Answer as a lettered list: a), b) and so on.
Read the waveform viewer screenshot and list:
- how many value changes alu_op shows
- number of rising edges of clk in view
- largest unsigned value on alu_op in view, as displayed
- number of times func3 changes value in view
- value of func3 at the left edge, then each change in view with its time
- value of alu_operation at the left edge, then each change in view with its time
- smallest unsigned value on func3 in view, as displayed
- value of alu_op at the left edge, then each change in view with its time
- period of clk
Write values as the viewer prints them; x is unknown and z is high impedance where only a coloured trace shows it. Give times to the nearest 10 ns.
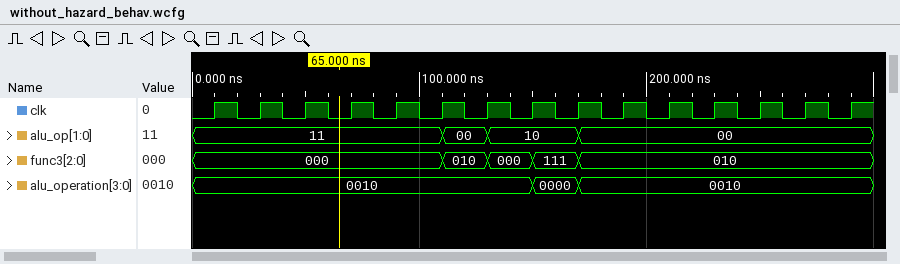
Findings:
a) 3
b) 15
c) 11
d) 4
e) 000, 010 at 110 ns, 000 at 130 ns, 111 at 150 ns, 010 at 170 ns
f) 0010, 0000 at 150 ns, 0010 at 170 ns
g) 000
h) 11, 00 at 110 ns, 10 at 130 ns, 00 at 170 ns
i) 20 ns
